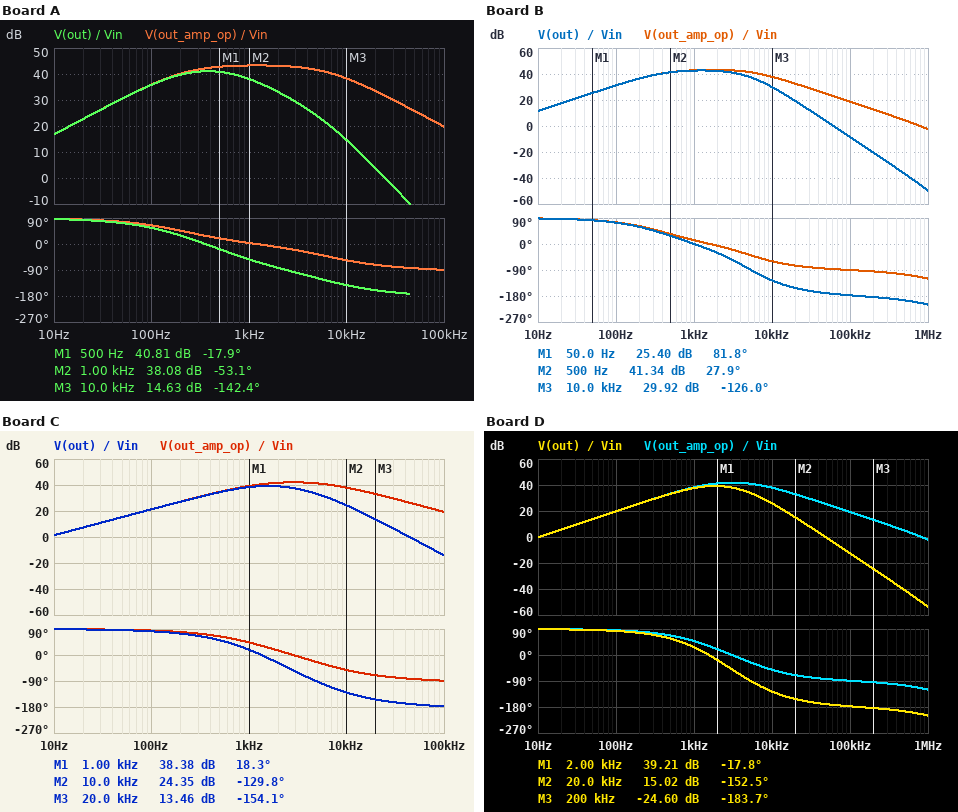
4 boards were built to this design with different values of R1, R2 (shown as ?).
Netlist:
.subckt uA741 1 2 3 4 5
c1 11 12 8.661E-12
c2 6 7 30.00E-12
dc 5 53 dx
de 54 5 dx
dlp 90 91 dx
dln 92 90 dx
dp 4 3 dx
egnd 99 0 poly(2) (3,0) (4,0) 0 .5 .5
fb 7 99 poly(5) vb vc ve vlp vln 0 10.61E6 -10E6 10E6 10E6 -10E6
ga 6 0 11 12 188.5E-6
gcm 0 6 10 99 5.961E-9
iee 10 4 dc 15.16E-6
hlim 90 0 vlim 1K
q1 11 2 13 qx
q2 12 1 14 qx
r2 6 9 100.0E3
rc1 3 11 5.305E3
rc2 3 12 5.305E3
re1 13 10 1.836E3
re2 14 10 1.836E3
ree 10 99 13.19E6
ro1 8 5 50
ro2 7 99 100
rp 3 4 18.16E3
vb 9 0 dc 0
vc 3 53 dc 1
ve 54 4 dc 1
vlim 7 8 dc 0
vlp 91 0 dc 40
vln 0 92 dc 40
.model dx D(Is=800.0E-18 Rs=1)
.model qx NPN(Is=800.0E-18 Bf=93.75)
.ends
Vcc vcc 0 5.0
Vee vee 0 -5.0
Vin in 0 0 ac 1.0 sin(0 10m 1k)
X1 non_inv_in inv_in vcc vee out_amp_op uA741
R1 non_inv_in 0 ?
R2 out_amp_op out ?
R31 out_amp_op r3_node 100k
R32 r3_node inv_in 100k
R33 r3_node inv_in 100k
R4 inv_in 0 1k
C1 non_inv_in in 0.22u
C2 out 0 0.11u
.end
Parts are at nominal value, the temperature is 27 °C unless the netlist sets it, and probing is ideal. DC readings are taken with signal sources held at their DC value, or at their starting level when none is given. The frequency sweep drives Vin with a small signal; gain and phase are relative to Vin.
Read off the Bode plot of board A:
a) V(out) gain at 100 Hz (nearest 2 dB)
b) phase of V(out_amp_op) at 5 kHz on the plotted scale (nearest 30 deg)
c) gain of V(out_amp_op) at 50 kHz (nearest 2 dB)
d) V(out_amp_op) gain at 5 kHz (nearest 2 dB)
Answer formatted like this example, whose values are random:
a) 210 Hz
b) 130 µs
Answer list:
a) 36 dB
b) -30 deg
c) 26 dB
d) 42 dB
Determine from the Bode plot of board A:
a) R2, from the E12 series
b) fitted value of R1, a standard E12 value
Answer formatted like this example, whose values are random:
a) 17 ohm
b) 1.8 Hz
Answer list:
a) 2.2 kΩ
b) 3.3 kΩ
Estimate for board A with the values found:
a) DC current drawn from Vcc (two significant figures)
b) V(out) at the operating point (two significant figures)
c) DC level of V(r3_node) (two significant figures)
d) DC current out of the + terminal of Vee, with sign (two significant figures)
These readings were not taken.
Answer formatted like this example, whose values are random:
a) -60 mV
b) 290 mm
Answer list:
a) 570 µA
b) -25 mV
c) -8.4 mV
d) -570 µA
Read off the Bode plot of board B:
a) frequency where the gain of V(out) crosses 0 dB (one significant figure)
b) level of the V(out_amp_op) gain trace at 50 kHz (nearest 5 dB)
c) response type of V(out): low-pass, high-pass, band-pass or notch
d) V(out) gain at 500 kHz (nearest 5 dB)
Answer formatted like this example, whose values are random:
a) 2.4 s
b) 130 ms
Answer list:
a) 60 kHz
b) 25 dB
c) band-pass
d) -35 dB
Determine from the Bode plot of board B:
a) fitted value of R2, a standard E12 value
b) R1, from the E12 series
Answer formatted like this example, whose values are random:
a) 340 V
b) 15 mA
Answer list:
a) 330 Ω
b) 1.8 kΩ
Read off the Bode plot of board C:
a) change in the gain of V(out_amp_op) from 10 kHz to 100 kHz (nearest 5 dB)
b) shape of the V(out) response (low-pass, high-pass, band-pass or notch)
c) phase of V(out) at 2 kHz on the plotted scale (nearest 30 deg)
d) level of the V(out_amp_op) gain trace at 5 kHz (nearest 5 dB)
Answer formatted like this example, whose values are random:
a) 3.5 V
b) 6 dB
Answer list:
a) -20 dB
b) band-pass
c) -30 deg
d) 40 dB
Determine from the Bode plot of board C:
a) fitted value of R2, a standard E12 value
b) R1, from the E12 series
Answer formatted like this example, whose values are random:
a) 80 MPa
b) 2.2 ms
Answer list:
a) 680 Ω
b) 560 Ω
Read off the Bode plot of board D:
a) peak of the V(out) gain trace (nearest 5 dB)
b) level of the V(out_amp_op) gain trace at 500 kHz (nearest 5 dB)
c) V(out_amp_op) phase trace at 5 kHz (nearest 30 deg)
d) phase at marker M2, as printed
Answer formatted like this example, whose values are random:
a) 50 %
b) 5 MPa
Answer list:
a) 40 dB
b) 5 dB
c) -30 deg
d) -152.5 deg
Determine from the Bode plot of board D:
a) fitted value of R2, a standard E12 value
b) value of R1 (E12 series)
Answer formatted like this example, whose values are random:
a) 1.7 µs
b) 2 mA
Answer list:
a) 560 Ω
b) 470 Ω
